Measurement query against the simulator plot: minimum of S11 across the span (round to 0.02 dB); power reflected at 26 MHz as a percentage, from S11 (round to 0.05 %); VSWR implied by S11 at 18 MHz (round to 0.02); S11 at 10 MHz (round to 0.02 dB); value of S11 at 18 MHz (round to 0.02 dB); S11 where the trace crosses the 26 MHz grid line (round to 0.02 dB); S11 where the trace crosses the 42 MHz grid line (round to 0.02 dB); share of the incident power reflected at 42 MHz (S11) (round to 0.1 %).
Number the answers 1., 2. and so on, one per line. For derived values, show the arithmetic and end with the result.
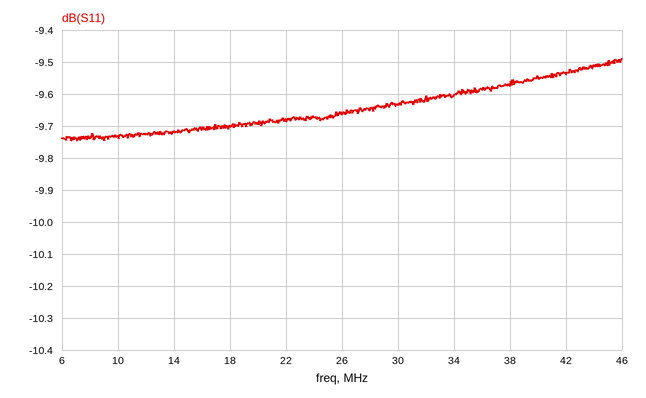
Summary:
1. -9.74 dB
2. 10^(-9.66/10) ≈ 10.80 %
3. |Γ| = 10^(-9.7/20) = 0.3273; VSWR = (1 + 0.3273)/(1 − 0.3273) ≈ 1.97, so 1.98 to the nearest 0.02
4. -9.74 dB
5. -9.70 dB
6. -9.66 dB
7. -9.54 dB
8. 10^(-9.54/10) ≈ 11.1 %
